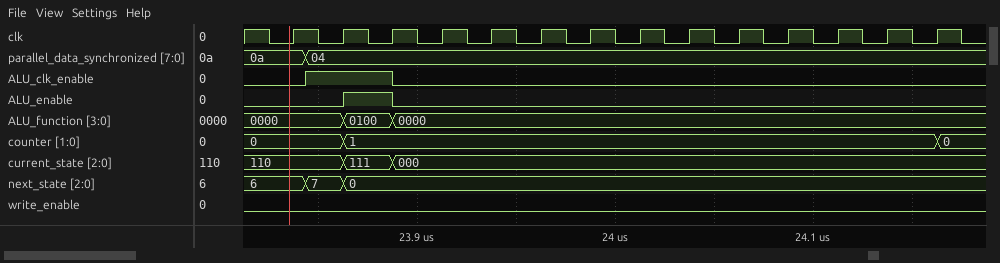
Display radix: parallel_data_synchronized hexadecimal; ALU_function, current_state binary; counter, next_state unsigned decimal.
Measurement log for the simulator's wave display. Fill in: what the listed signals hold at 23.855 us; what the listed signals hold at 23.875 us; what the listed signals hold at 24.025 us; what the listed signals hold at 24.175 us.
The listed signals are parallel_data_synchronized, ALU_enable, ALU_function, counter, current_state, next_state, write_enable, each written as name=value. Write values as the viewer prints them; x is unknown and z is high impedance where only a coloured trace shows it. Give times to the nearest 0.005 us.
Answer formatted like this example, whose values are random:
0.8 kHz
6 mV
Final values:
parallel_data_synchronized=04, ALU_enable=0, ALU_function=0000, counter=0, current_state=110, next_state=7, write_enable=0
parallel_data_synchronized=04, ALU_enable=1, ALU_function=0100, counter=1, current_state=111, next_state=0, write_enable=0
parallel_data_synchronized=04, ALU_enable=0, ALU_function=0000, counter=1, current_state=000, next_state=0, write_enable=0
parallel_data_synchronized=04, ALU_enable=0, ALU_function=0000, counter=0, current_state=000, next_state=0, write_enable=0
